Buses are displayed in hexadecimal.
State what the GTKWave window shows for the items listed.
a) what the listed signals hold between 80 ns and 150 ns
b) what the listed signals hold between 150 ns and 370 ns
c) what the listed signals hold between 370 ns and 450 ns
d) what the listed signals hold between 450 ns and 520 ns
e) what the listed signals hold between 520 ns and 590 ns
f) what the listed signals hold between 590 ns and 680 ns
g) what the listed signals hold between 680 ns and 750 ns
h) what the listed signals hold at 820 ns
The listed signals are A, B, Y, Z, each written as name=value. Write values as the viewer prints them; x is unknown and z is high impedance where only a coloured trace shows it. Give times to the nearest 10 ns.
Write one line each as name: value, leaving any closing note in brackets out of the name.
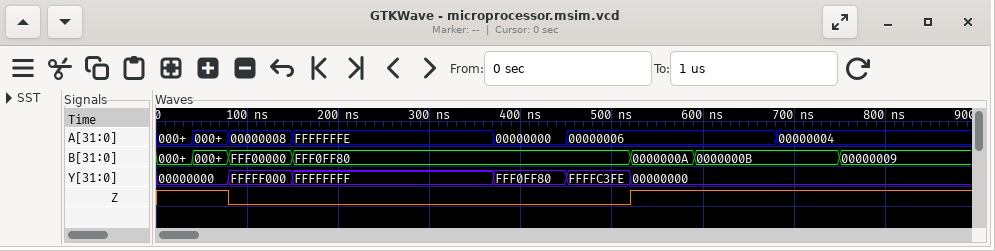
what the listed signals hold between 80 ns and 150 ns: A=00000008, B=FFF00000, Y=FFFFF000, Z=0
what the listed signals hold between 150 ns and 370 ns: A=FFFFFFFE, B=FFF0FF80, Y=FFFFFFFF, Z=0
what the listed signals hold between 370 ns and 450 ns: A=00000000, B=FFF0FF80, Y=FFF0FF80, Z=0
what the listed signals hold between 450 ns and 520 ns: A=00000006, B=FFF0FF80, Y=FFFFC3FE, Z=0
what the listed signals hold between 520 ns and 590 ns: A=00000006, B=0000000A, Y=00000000, Z=1
what the listed signals hold between 590 ns and 680 ns: A=00000006, B=0000000B, Y=00000000, Z=1
what the listed signals hold between 680 ns and 750 ns: A=00000004, B=0000000B, Y=00000000, Z=1
what the listed signals hold at 820 ns: A=00000004, B=00000009, Y=00000000, Z=1
